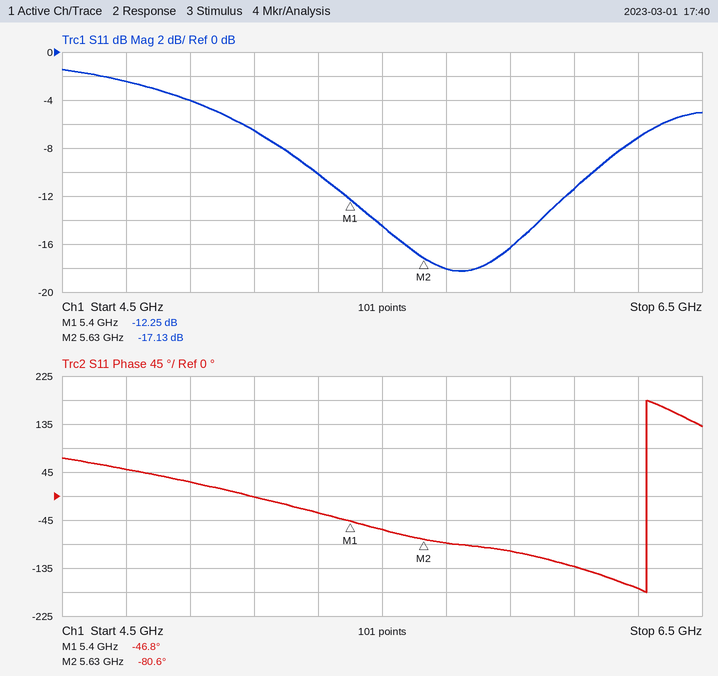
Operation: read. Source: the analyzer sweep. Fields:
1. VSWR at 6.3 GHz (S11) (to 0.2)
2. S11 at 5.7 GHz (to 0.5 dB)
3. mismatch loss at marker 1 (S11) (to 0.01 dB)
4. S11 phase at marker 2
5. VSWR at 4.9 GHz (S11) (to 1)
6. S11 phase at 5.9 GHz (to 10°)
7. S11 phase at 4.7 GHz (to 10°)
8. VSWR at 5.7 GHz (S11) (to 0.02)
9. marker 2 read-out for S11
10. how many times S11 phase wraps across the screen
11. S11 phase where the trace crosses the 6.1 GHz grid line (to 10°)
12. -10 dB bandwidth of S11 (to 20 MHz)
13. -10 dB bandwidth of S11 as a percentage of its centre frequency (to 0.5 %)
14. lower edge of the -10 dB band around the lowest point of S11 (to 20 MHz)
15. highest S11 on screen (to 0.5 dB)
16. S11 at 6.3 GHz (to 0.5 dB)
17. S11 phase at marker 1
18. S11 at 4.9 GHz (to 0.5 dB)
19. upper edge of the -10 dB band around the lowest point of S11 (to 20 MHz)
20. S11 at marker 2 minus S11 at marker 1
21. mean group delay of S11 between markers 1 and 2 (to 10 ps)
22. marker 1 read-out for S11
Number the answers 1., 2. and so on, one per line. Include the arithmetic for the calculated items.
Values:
1. |Γ| = 10^(-7/20) = 0.4467; VSWR = (1 + 0.4467)/(1 − 0.4467) ≈ 2.6
2. -18.0 dB
3. −10 log10(1 − 10^(-12.25/10)) ≈ 0.27 dB
4. -80.6°
5. |Γ| = 10^(-4/20) = 0.6310; VSWR = (1 + 0.6310)/(1 − 0.6310) ≈ 4
6. -100°
7. 50°
8. |Γ| = 10^(-18/20) = 0.1259; VSWR = (1 + 0.1259)/(1 − 0.1259) ≈ 1.29, so 1.28 to the nearest 0.02
9. -17.13 dB
10. 1
11. -130°
12. 6.16 GHz − 5.30 GHz = 860 MHz
13. 860 MHz / 5.73 GHz ≈ 15.0 %
14. 5.30 GHz
15. -1.5 dB
16. -7.0 dB
17. -46.8°
18. -4.0 dB
19. 6.16 GHz
20. -17.13 − (-12.25) = -4.88 dB
21. −(-80.6° − (-46.8°))/(360° × 230 MHz) ≈ 408 ps, so 410 ps to the nearest 10 ps
22. -12.25 dB
